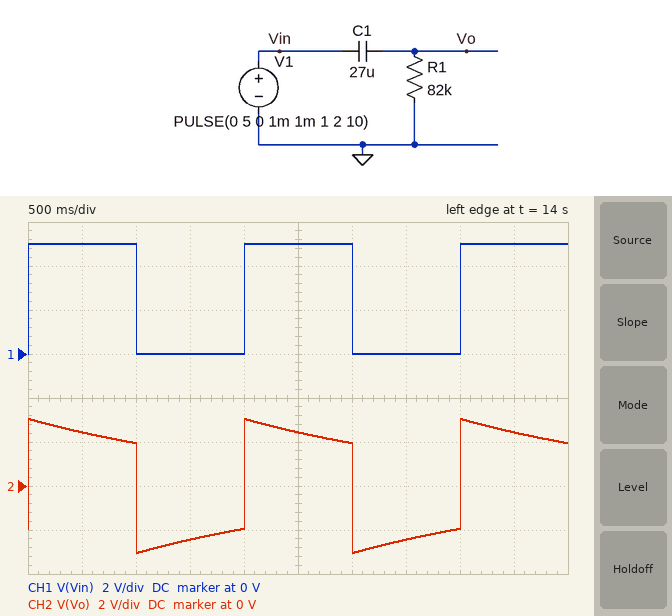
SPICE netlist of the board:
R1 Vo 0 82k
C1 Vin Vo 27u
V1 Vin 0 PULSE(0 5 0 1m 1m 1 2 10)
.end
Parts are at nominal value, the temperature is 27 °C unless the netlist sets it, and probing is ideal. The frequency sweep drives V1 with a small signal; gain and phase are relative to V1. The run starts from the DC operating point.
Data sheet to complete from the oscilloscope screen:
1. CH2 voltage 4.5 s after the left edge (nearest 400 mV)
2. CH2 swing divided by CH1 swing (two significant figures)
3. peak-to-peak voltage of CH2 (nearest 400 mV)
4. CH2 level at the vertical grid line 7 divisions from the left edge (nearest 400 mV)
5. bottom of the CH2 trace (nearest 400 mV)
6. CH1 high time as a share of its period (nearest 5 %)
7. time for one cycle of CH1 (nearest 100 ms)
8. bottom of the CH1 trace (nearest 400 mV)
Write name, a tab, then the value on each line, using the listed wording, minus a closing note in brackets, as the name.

CH2 voltage 4.5 s after the left edge	2.4 V
CH2 swing divided by CH1 swing	1.2
peak-to-peak voltage of CH2	6.0 V
CH2 level at the vertical grid line 7 divisions from the left edge	-2.4 V
bottom of the CH2 trace	-3.2 V
CH1 high time as a share of its period	50 %
time for one cycle of CH1	2.0 s
bottom of the CH1 trace	0 V
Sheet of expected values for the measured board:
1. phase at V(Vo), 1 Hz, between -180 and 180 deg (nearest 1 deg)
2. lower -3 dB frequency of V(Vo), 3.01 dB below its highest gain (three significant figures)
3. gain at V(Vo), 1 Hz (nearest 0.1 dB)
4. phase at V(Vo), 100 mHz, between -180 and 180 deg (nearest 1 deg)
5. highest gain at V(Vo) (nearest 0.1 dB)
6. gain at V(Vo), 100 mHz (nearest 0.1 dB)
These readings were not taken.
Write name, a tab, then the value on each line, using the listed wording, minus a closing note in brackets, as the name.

phase at V(Vo), 1 Hz, between -180 and 180 deg	4 deg
lower -3 dB frequency of V(Vo), 3.01 dB below its highest gain	71.9 mHz
gain at V(Vo), 1 Hz	0 dB
phase at V(Vo), 100 mHz, between -180 and 180 deg	36 deg
highest gain at V(Vo)	0 dB
gain at V(Vo), 100 mHz	-1.8 dB
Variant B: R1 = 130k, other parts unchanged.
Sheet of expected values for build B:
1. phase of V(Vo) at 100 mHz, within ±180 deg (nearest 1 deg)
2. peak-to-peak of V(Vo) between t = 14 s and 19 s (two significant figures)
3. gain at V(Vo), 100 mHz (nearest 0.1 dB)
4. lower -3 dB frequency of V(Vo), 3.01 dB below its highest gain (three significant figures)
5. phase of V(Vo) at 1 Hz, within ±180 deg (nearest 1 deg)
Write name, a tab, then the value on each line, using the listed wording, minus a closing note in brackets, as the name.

phase of V(Vo) at 100 mHz, within ±180 deg	24 deg
peak-to-peak of V(Vo) between t = 14 s and 19 s	5.7 V
gain at V(Vo), 100 mHz	-0.8 dB
lower -3 dB frequency of V(Vo), 3.01 dB below its highest gain	45.3 mHz
phase of V(Vo) at 1 Hz, within ±180 deg	3 deg
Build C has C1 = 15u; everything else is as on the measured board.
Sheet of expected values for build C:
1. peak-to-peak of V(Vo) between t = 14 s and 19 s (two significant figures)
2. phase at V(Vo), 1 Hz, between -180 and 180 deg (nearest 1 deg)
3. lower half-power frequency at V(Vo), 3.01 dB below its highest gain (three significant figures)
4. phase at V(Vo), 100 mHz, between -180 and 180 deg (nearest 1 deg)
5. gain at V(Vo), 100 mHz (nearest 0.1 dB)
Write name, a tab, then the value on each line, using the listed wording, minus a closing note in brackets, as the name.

peak-to-peak of V(Vo) between t = 14 s and 19 s	6.9 V
phase at V(Vo), 1 Hz, between -180 and 180 deg	7 deg
lower half-power frequency at V(Vo), 3.01 dB below its highest gain	129 mHz
phase at V(Vo), 100 mHz, between -180 and 180 deg	52 deg
gain at V(Vo), 100 mHz	-4.3 dB
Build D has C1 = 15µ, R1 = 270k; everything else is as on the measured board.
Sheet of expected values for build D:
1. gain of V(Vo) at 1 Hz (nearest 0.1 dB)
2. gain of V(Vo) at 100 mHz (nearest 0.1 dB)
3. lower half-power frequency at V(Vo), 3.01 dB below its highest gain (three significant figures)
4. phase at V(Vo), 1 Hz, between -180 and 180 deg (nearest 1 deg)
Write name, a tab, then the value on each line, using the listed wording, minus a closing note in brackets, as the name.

gain of V(Vo) at 1 Hz	0 dB
gain of V(Vo) at 100 mHz	-0.6 dB
lower half-power frequency at V(Vo), 3.01 dB below its highest gain	39.3 mHz
phase at V(Vo), 1 Hz, between -180 and 180 deg	2 deg
